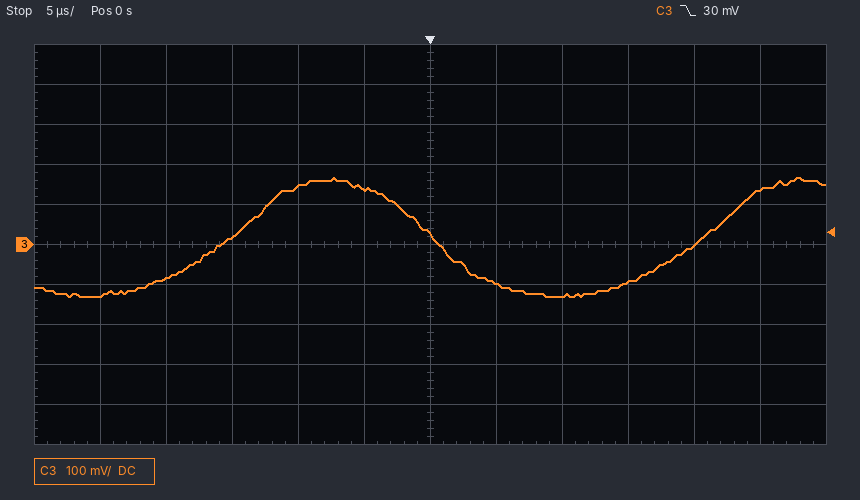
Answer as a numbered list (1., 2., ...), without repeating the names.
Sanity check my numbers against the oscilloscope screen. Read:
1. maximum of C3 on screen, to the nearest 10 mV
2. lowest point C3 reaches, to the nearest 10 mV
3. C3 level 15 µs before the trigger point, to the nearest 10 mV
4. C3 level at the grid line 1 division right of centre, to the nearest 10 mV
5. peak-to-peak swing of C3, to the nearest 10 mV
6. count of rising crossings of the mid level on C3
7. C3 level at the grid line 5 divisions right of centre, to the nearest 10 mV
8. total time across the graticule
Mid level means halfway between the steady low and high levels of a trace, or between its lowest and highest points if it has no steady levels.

1. 170 mV
2. -130 mV
3. 20 mV
4. -100 mV
5. 300 mV
6. 2
7. 140 mV
8. 60 µs
